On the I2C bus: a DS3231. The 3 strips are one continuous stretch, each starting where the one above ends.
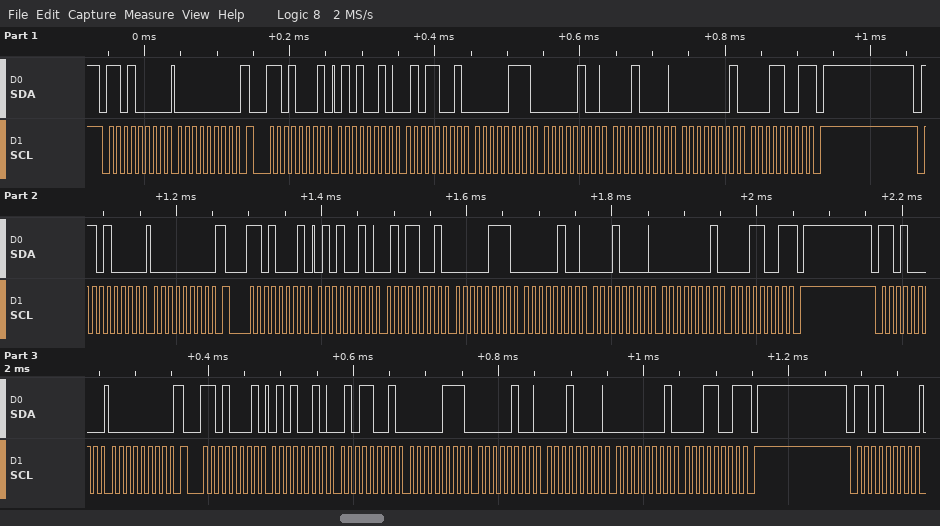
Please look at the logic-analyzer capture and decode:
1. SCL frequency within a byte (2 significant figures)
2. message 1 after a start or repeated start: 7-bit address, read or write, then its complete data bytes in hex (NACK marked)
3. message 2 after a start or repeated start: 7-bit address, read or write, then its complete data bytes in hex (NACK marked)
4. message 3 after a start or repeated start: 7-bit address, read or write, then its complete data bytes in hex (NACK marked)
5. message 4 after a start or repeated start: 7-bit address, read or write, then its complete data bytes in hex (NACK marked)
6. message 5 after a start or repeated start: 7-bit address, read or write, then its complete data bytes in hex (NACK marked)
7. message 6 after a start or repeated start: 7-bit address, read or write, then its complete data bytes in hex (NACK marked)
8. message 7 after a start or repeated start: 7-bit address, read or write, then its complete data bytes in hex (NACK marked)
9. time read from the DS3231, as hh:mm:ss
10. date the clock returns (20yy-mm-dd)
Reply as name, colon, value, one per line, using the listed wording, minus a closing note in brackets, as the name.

SCL frequency within a byte: 100 kHz
message 1 after a start or repeated start: 7-bit address, read or write, then its complete data bytes in hex: 0x68 write: 00
message 2 after a start or repeated start: 7-bit address, read or write, then its complete data bytes in hex: 0x68 read: 52 59 07 04 10 01 19 NACK
message 3 after a start or repeated start: 7-bit address, read or write, then its complete data bytes in hex: 0x68 write: 00
message 4 after a start or repeated start: 7-bit address, read or write, then its complete data bytes in hex: 0x68 read: 52 59 07 04 10 01 19 NACK
message 5 after a start or repeated start: 7-bit address, read or write, then its complete data bytes in hex: 0x68 write: 00
message 6 after a start or repeated start: 7-bit address, read or write, then its complete data bytes in hex: 0x68 read: 52 59 07 04 10 01 19 NACK
message 7 after a start or repeated start: 7-bit address, read or write, then its complete data bytes in hex: 0x68 write
time read from the DS3231, as hh:mm:ss: 07:59:52
date the clock returns: 2019-01-10
